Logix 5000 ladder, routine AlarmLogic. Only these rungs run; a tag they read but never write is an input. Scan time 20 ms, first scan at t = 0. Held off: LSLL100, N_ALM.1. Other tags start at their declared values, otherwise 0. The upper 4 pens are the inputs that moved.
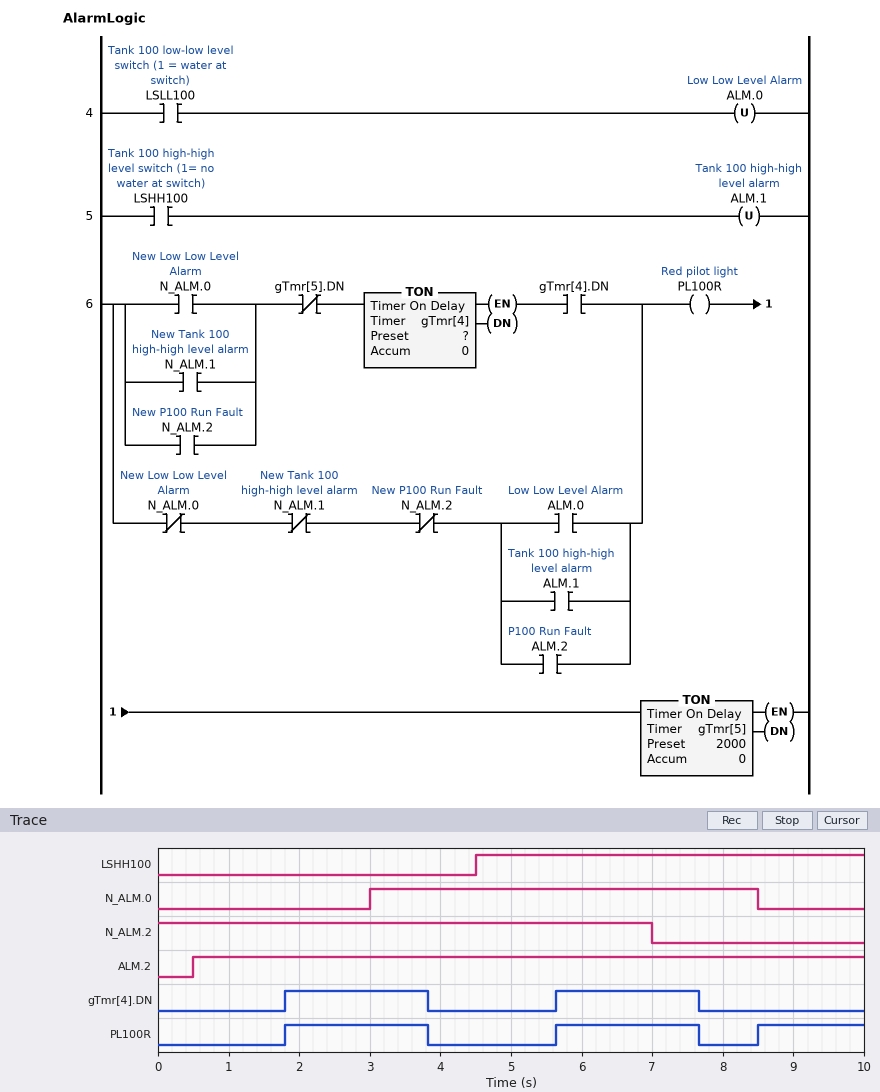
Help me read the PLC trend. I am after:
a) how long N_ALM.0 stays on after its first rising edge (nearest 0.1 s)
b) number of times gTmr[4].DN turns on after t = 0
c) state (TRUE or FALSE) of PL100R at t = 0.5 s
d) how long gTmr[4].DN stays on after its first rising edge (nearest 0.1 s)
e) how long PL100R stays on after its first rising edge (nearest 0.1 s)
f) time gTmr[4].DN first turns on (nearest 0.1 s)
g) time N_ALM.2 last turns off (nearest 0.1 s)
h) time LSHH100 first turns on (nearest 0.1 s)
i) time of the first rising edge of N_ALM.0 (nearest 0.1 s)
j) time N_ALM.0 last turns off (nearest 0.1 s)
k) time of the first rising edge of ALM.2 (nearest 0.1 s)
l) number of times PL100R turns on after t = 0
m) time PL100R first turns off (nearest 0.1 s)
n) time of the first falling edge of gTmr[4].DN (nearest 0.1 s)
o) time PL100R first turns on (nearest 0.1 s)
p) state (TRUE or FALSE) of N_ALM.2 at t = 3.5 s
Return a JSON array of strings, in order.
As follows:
["5.5 s", "2", "FALSE", "2.0 s", "2.0 s", "1.8 s", "7.0 s", "4.5 s", "3.0 s", "8.5 s", "0.5 s", "3", "3.8 s", "3.8 s", "1.8 s", "TRUE"]
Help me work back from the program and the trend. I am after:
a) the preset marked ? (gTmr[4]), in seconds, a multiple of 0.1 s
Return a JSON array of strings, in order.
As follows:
["1.8 s"]
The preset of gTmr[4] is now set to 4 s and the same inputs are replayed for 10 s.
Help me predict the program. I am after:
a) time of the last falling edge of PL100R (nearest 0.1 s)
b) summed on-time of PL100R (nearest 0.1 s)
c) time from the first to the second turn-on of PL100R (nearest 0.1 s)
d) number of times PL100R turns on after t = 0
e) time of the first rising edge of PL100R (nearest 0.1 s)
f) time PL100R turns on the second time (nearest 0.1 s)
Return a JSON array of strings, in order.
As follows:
["6.0 s", "3.5 s", "4.5 s", "2", "4.0 s", "8.5 s"]
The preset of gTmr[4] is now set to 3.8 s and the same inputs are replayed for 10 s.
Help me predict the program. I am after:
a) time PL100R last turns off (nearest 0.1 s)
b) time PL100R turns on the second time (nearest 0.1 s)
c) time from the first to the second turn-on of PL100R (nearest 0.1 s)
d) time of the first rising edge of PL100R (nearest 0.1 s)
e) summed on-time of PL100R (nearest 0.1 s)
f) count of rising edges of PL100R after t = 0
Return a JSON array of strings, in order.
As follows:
["5.8 s", "8.5 s", "4.7 s", "3.8 s", "3.5 s", "2"]
